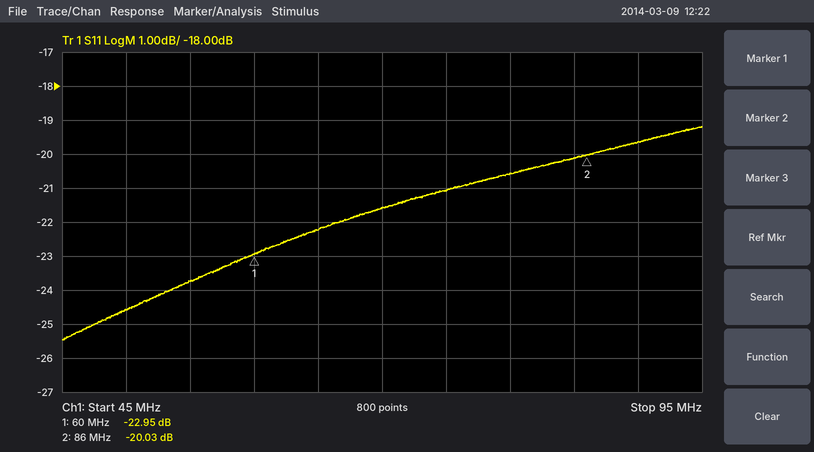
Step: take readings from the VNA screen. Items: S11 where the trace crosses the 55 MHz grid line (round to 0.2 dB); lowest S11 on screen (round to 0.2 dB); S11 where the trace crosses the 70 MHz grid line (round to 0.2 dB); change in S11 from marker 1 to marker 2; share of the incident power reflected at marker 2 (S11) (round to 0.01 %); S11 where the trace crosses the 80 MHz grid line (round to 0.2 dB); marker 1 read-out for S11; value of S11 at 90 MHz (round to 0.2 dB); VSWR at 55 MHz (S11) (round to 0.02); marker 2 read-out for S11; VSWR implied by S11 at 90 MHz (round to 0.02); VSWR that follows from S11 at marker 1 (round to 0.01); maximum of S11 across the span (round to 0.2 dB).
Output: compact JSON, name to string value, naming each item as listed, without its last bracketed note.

{"S11 where the trace crosses the 55 MHz grid line": "-23.8 dB", "lowest S11 on screen": "-25.4 dB", "S11 where the trace crosses the 70 MHz grid line": "-21.6 dB", "change in S11 from marker 1 to marker 2": "2.92 dB", "share of the incident power reflected at marker 2 (S11)": "0.99 %", "S11 where the trace crosses the 80 MHz grid line": "-20.6 dB", "marker 1 read-out for S11": "-22.95 dB", "value of S11 at 90 MHz": "-19.6 dB", "VSWR at 55 MHz (S11)": "1.14", "marker 2 read-out for S11": "-20.03 dB", "VSWR implied by S11 at 90 MHz": "1.24", "VSWR that follows from S11 at marker 1": "1.15", "maximum of S11 across the span": "-19.2 dB"}
